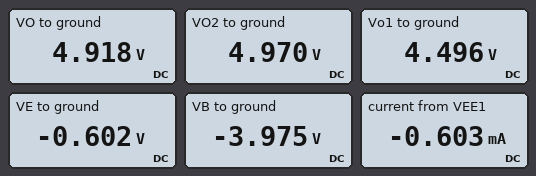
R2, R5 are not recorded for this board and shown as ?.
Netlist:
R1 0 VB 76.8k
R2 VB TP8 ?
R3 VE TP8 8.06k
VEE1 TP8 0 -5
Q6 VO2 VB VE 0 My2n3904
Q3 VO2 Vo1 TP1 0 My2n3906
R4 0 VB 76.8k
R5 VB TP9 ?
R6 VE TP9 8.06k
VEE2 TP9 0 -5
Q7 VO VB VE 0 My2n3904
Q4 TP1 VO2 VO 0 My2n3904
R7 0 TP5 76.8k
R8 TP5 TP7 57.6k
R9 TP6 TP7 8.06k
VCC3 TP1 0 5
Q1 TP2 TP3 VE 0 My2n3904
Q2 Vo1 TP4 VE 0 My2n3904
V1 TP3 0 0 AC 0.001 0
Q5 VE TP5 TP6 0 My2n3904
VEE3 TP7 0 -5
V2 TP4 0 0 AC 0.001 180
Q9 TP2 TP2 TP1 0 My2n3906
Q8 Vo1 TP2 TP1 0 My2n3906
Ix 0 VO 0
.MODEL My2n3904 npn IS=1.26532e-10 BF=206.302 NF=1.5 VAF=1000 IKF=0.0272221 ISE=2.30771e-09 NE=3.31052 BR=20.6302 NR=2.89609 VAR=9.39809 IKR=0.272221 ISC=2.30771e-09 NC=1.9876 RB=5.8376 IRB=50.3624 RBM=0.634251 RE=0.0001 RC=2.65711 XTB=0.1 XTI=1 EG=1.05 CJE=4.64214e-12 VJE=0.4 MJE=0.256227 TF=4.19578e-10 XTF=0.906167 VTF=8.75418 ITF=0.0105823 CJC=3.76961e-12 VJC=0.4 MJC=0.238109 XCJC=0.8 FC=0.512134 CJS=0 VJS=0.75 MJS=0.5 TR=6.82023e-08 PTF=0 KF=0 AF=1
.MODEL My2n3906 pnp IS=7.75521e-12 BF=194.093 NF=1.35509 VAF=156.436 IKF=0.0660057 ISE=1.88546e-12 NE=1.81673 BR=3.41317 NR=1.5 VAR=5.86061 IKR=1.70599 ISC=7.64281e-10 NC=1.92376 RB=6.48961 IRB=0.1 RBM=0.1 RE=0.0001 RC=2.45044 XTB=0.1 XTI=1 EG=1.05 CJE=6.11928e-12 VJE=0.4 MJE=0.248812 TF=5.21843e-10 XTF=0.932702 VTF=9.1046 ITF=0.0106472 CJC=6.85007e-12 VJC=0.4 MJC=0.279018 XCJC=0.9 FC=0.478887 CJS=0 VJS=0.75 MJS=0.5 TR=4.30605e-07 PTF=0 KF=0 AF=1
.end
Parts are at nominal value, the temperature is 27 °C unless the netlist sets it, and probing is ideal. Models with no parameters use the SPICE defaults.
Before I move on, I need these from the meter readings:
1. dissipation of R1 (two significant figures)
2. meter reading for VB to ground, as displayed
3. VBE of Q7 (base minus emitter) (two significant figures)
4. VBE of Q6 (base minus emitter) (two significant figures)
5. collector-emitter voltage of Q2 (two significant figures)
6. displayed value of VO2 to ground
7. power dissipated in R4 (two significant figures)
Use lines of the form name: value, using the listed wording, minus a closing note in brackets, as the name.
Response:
dissipation of R1: 210 µW
meter reading for VB to ground, as displayed: -3.975 V
VBE of Q7 (base minus emitter): -3.4 V
VBE of Q6 (base minus emitter): -3.4 V
collector-emitter voltage of Q2: 5.1 V
displayed value of VO2 to ground: 4.970 V
power dissipated in R4: 210 µW
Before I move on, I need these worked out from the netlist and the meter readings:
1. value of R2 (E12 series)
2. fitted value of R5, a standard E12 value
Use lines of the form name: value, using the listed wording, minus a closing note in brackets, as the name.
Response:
value of R2: 18 kΩ
fitted value of R5, a standard E12 value: 22 kΩ
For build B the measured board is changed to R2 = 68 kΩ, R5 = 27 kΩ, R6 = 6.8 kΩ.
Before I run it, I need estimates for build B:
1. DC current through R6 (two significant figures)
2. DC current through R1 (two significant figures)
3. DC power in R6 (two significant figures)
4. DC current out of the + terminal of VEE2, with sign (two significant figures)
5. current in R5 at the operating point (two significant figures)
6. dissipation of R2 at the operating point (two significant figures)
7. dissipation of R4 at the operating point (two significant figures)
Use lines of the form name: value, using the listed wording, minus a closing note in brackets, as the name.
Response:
DC current through R6: 650 µA
DC current through R1: 43 µA
DC power in R6: 2.8 mW
DC current out of the + terminal of VEE2, with sign: -710 µA
current in R5 at the operating point: 62 µA
dissipation of R2 at the operating point: 41 µW
dissipation of R4 at the operating point: 140 µW
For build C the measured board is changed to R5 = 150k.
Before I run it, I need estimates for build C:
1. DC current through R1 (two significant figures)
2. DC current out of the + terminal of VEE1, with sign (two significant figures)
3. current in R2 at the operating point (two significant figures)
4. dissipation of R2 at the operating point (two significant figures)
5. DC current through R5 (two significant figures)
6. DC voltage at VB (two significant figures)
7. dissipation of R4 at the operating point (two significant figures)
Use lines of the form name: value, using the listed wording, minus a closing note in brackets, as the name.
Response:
DC current through R1: 46 µA
DC current out of the + terminal of VEE1, with sign: -630 µA
current in R2 at the operating point: 82 µA
dissipation of R2 at the operating point: 120 µW
DC current through R5: 9.8 µA
DC voltage at VB: -3.5 V
dissipation of R4 at the operating point: 160 µW
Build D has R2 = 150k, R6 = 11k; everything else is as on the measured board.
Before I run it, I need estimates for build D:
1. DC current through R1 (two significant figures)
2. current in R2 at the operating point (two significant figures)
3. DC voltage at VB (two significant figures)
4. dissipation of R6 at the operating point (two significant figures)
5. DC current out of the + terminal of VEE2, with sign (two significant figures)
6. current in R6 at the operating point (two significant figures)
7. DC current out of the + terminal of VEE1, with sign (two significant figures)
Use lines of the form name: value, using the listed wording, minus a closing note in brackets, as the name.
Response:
DC current through R1: 43 µA
current in R2 at the operating point: 11 µA
DC voltage at VB: -3.3 V
dissipation of R6 at the operating point: 1.8 mW
DC current out of the + terminal of VEE2, with sign: -480 µA
current in R6 at the operating point: 400 µA
DC current out of the + terminal of VEE1, with sign: -560 µA
